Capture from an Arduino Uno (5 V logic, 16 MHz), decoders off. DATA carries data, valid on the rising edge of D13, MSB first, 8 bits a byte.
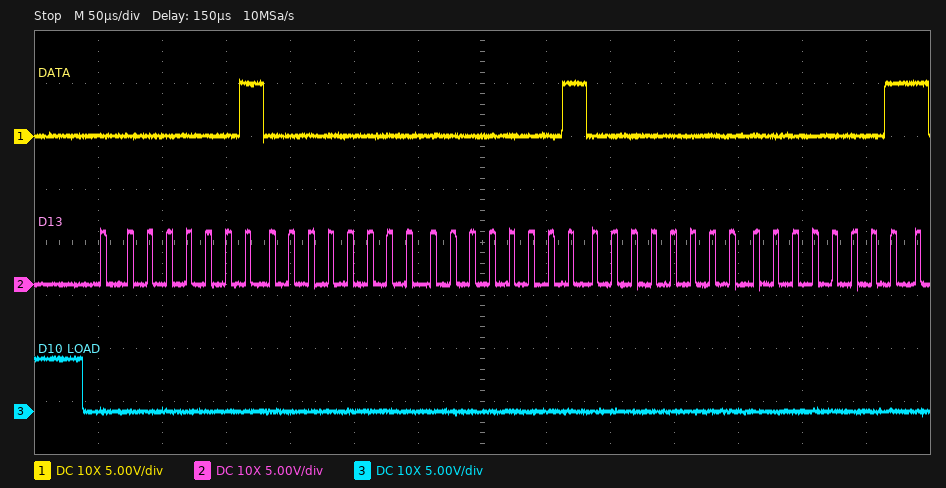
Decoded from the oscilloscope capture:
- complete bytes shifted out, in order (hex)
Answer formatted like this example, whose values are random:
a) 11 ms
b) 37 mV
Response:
a) 01 00 01 00 01
